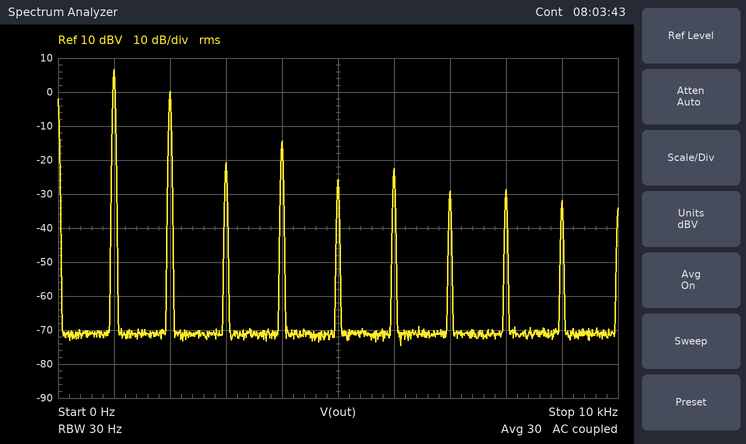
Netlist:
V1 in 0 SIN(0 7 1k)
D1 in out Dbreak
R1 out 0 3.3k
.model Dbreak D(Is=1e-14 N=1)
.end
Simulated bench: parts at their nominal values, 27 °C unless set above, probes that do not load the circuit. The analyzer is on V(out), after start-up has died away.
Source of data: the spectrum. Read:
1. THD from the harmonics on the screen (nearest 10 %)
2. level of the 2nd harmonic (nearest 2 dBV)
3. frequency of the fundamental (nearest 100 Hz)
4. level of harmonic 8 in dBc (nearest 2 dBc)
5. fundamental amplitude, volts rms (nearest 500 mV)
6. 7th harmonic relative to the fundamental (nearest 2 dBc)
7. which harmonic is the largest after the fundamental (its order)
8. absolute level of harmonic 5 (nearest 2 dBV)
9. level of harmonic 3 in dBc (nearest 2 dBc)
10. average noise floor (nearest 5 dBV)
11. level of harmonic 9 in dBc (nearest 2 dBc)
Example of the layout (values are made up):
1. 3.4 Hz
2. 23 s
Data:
1. 50 %
2. 0 dBV
3. 1.0 kHz
4. -36 dBc
5. 2.0 V
6. -36 dBc
7. 2
8. -26 dBV
9. -28 dBc
10. -70 dBV
11. -38 dBc
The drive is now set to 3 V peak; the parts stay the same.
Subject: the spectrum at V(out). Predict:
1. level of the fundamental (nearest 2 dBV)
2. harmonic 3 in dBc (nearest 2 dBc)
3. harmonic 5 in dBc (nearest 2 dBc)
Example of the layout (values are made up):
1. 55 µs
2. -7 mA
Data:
1. -2 dBV
2. -20 dBc
3. -26 dBc
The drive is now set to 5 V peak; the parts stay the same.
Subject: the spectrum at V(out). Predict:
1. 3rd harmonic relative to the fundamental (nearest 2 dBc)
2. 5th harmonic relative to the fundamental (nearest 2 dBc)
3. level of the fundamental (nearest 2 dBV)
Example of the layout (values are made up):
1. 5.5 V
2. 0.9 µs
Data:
1. -24 dBc
2. -30 dBc
3. 4 dBV
